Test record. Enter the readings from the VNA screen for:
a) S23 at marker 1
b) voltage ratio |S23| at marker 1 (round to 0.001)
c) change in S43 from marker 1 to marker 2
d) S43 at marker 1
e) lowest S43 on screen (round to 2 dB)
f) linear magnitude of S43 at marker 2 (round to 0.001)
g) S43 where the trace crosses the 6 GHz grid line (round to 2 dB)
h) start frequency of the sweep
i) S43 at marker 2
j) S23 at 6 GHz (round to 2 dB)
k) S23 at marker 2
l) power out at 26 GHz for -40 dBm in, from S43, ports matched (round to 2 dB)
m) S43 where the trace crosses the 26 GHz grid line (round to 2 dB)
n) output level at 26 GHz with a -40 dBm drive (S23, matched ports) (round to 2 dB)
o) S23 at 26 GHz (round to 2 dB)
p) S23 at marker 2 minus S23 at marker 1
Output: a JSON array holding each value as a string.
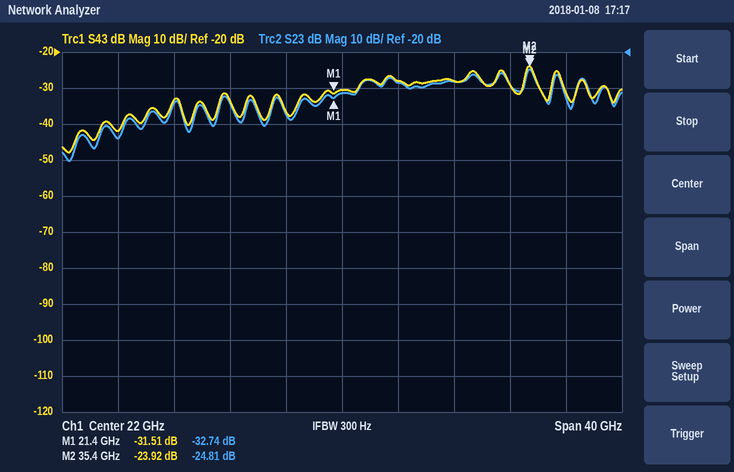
["-32.74 dB", "0.023", "7.59 dB", "-31.51 dB", "-48 dB", "0.064", "-42 dB", "2 GHz", "-23.92 dB", "-44 dB", "-24.81 dB", "-68 dBm", "-28 dB", "-68 dBm", "-28 dB", "7.93 dB"]
